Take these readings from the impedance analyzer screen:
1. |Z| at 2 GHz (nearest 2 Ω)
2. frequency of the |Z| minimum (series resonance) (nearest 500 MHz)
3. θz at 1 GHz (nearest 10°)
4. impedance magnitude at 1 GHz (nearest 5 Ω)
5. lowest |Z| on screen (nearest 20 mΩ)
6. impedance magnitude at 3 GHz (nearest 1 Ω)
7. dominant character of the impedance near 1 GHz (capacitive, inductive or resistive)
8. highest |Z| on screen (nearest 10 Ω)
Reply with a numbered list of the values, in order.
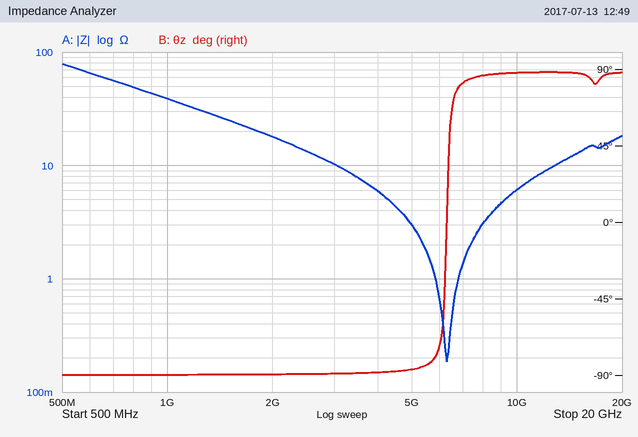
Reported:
1. 18 Ω
2. 6.5 GHz
3. -90°
4. 40 Ω
5. 180 mΩ
6. 10 Ω
7. capacitive
8. 80 Ω
